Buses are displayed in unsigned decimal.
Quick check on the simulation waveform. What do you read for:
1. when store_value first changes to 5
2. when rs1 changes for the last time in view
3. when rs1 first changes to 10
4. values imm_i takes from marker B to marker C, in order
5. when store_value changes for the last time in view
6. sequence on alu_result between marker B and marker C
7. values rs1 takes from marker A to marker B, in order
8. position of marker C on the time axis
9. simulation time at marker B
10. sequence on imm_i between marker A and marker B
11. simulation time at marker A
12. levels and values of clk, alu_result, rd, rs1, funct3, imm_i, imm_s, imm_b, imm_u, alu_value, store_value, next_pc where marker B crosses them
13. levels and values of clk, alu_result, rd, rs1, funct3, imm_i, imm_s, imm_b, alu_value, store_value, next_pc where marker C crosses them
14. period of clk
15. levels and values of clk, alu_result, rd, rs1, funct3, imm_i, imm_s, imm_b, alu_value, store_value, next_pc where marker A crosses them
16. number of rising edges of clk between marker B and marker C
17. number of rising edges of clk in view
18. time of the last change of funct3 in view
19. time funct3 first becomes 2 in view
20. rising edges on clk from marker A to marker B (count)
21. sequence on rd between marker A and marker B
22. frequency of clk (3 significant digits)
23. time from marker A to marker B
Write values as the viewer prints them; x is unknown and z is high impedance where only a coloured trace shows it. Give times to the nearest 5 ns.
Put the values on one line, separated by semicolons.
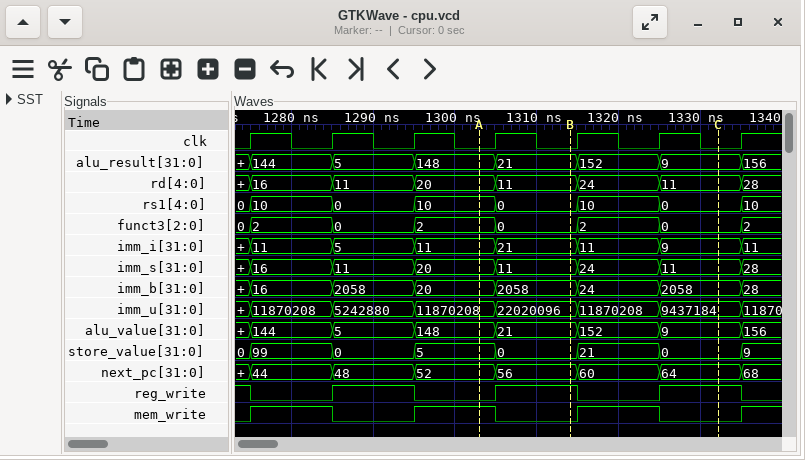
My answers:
1295 ns; 1335 ns; 1275 ns; 21, 11, 9; 1335 ns; 21, 152, 9; 10, 0; 1330 ns; 1315 ns; 11, 21; 1305 ns; clk=0, alu_result=21, rd=11, rs1=0, funct3=0, imm_i=21, imm_s=11, imm_b=2058, imm_u=22020096, alu_value=21, store_value=0, next_pc=56; clk=0, alu_result=9, rd=11, rs1=0, funct3=0, imm_i=9, imm_s=11, imm_b=2058, alu_value=9, store_value=0, next_pc=64; 10 ns; clk=0, alu_result=148, rd=20, rs1=10, funct3=2, imm_i=11, imm_s=20, imm_b=20, alu_value=148, store_value=5, next_pc=52; 2; 7; 1335 ns; 1275 ns; 1; 20, 11; 100 MHz; 10 ns
